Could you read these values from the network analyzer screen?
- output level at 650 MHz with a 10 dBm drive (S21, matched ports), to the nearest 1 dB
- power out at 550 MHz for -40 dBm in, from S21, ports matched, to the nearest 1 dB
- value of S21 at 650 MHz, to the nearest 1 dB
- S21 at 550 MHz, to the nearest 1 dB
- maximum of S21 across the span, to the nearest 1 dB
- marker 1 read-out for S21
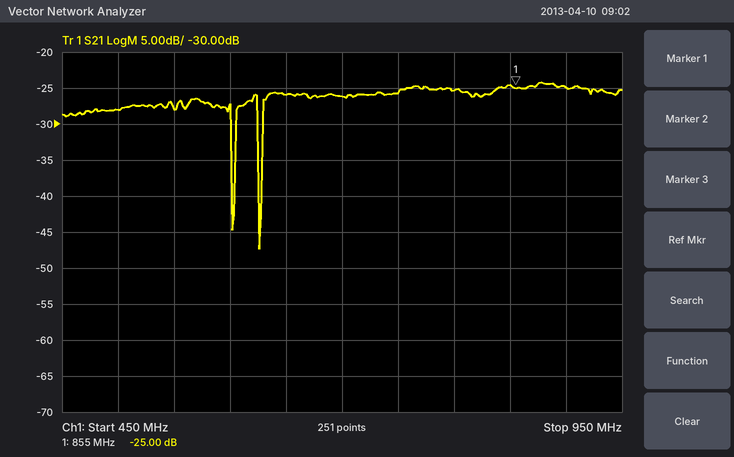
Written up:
-16 dBm
-68 dBm
-26 dB
-28 dB
-24 dB
-25.00 dB
